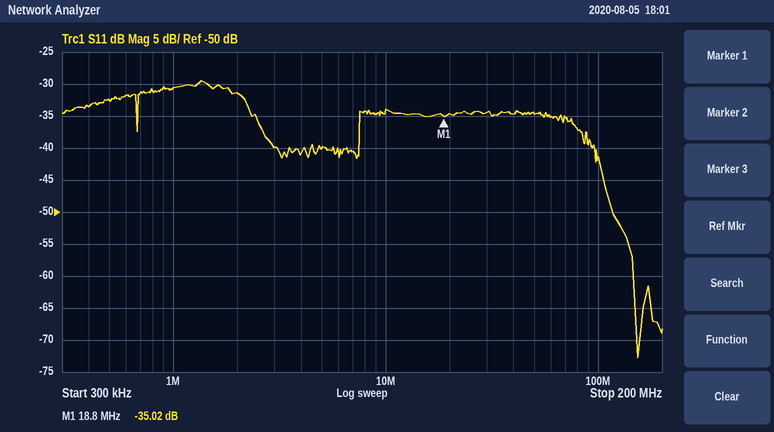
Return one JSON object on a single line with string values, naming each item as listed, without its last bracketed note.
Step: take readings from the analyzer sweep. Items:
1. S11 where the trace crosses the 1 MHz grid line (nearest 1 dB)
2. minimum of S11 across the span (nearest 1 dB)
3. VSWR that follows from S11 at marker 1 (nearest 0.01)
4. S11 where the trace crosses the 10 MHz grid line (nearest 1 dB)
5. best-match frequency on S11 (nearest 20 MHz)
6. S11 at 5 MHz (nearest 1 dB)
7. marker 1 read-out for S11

{"S11 where the trace crosses the 1 MHz grid line": "-31 dB", "minimum of S11 across the span": "-73 dB", "VSWR that follows from S11 at marker 1": "1.04", "S11 where the trace crosses the 10 MHz grid line": "-34 dB", "best-match frequency on S11": "160 MHz", "S11 at 5 MHz": "-40 dB", "marker 1 read-out for S11": "-35.02 dB"}
